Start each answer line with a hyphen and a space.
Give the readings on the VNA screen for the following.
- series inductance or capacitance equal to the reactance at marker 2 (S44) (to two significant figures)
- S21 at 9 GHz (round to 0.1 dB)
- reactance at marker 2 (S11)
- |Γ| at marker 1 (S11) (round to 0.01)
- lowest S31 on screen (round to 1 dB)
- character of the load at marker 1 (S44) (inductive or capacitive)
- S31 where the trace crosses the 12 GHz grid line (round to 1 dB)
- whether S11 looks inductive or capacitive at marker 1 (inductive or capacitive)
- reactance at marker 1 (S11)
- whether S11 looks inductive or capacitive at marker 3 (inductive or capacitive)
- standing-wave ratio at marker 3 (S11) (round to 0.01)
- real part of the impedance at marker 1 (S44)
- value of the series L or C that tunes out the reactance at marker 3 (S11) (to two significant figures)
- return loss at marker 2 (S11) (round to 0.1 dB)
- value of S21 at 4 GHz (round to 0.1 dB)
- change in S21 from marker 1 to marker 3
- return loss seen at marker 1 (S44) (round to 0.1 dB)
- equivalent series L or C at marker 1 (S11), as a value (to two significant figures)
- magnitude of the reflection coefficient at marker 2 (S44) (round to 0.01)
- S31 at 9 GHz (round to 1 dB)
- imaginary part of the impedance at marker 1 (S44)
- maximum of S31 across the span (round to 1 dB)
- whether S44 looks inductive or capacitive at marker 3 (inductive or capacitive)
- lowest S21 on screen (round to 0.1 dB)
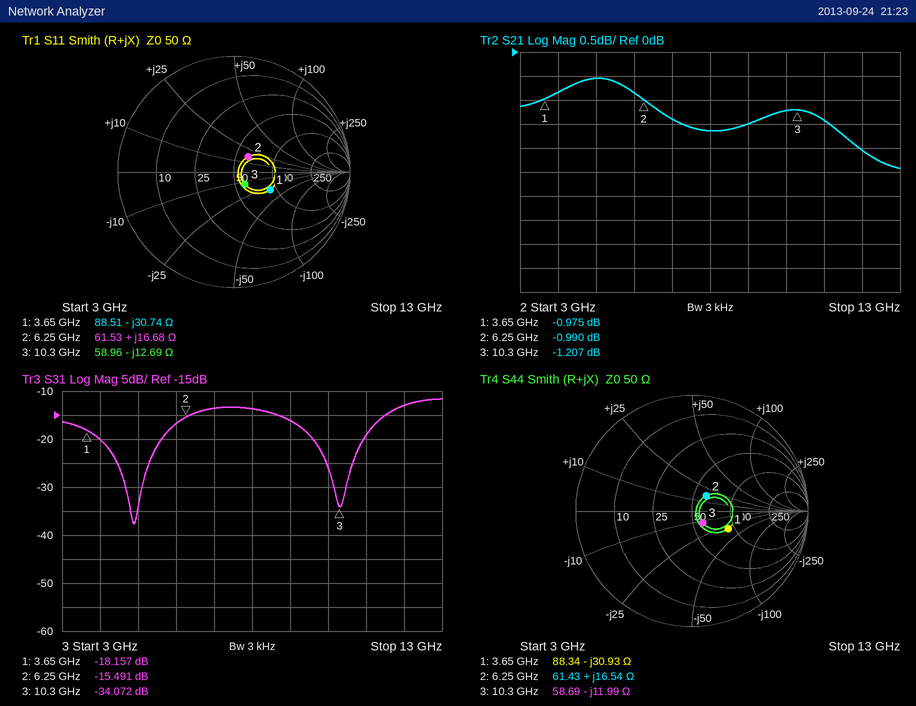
- 420 pH
- -1.5 dB
- +16.68 Ω
- 0.35
- -38 dB
- capacitive
- -13 dB
- capacitive
- -30.74 Ω
- capacitive
- 1.33
- 88.34 Ω
- 200 pH
- 14.9 dB
- -0.8 dB
- -0.232 dB
- 9.2 dB
- 1.4 pF
- 0.18
- -16 dB
- -30.93 Ω
- -12 dB
- capacitive
- -2.4 dB
